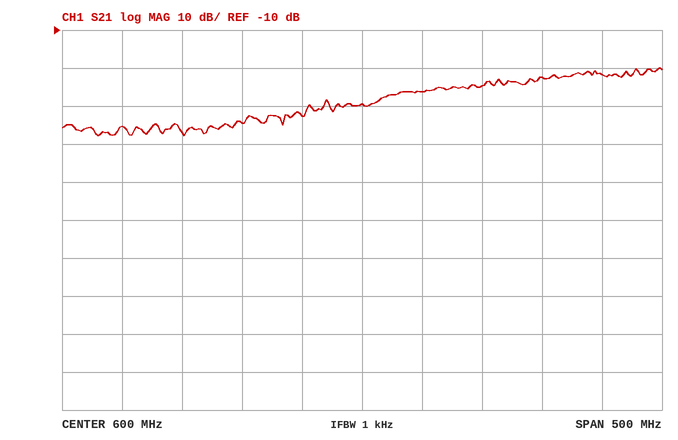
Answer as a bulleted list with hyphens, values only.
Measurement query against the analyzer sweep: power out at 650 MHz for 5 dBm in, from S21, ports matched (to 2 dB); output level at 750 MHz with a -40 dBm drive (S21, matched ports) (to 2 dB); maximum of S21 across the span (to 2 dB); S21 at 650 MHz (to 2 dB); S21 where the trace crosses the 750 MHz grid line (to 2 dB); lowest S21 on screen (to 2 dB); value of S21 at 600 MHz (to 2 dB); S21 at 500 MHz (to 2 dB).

- -22 dBm
- -62 dBm
- -20 dB
- -26 dB
- -22 dB
- -38 dB
- -30 dB
- -34 dB
